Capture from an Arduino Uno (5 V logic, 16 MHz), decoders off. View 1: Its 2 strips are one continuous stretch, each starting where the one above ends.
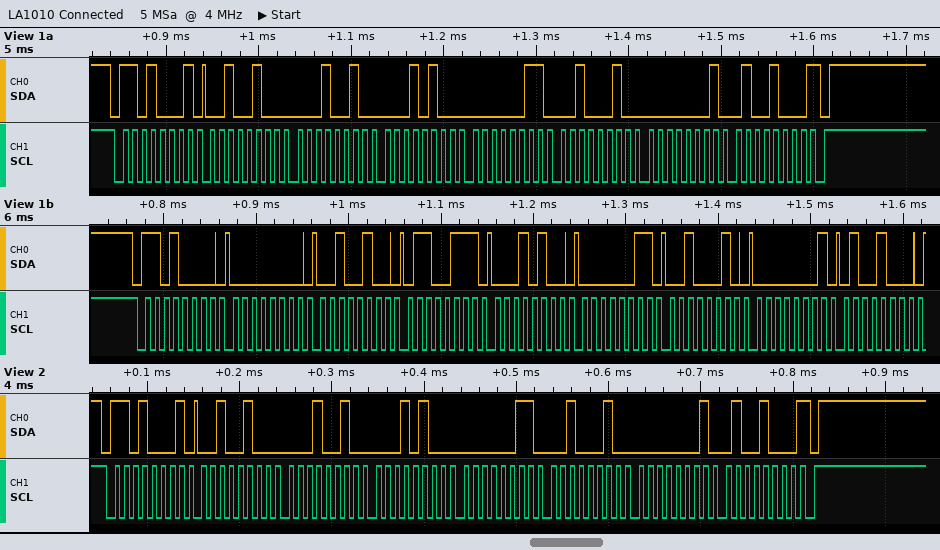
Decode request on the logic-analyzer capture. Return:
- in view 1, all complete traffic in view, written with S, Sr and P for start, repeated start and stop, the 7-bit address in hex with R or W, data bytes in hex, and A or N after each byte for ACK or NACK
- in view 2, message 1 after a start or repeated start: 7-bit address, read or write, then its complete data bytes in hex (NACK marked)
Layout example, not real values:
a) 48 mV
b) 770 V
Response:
a) S 68R A 24 A 12 A 14 A 03 A 22 A 01 A 48 N P S 68W A 00 A 24 A 67 A 14 A 03 A 22 A 01 A 48 A
b) 0x68 read: 24 12 14 03 22 01 48 NACK
